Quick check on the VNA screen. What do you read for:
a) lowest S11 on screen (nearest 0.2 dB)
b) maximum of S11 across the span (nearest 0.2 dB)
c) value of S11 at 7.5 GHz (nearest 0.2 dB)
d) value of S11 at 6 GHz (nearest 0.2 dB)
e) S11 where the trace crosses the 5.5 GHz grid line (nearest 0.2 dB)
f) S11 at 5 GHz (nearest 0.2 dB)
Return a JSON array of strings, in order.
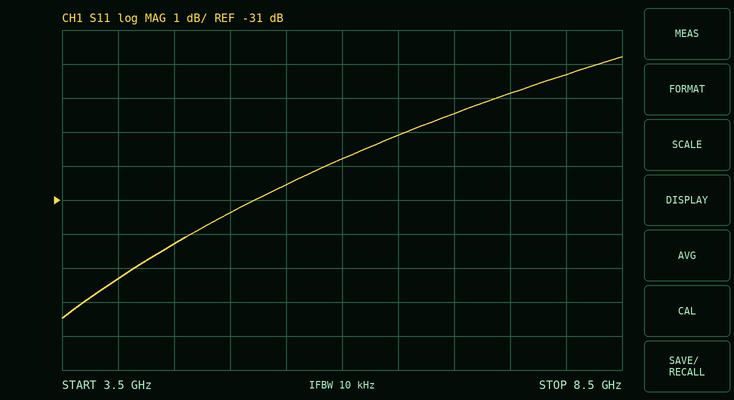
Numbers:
["-34.4 dB", "-26.8 dB", "-27.8 dB", "-29.8 dB", "-30.6 dB", "-31.4 dB"]
